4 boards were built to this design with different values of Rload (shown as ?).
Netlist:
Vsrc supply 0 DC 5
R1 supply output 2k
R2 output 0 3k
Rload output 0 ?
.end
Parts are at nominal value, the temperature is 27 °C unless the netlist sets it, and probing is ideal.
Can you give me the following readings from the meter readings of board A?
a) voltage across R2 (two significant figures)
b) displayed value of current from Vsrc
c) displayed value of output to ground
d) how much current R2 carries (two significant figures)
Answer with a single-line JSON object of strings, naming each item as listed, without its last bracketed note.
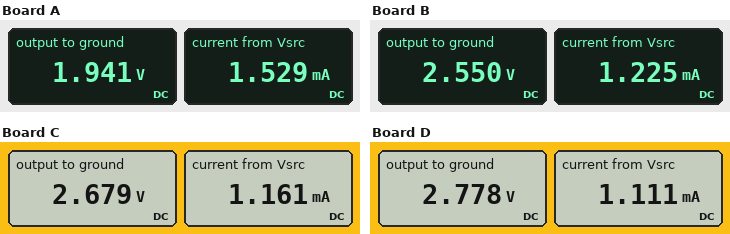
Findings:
{"voltage across R2": "1.9 V", "displayed value of current from Vsrc": "1.529 mA", "displayed value of output to ground": "1.941 V", "how much current R2 carries": "650 µA"}
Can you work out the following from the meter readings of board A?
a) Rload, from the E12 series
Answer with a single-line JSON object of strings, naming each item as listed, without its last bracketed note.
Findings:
{"Rload, from the E12 series": "2.2 kΩ"}
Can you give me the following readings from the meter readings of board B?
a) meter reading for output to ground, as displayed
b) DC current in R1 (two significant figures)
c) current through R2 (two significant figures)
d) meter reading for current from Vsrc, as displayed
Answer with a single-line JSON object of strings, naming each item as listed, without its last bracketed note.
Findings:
{"meter reading for output to ground, as displayed": "2.550 V", "DC current in R1": "1.2 mA", "current through R2": "850 µA", "meter reading for current from Vsrc, as displayed": "1.225 mA"}
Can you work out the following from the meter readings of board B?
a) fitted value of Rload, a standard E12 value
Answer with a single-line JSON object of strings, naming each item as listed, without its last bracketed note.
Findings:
{"fitted value of Rload, a standard E12 value": "6.8 kΩ"}
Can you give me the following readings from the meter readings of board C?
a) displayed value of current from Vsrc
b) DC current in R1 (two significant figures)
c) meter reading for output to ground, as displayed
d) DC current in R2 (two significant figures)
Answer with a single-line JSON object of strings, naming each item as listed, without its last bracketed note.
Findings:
{"displayed value of current from Vsrc": "1.161 mA", "DC current in R1": "1.2 mA", "meter reading for output to ground, as displayed": "2.679 V", "DC current in R2": "890 µA"}
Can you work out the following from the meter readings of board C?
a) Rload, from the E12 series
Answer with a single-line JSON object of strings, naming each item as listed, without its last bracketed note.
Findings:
{"Rload, from the E12 series": "10 kΩ"}
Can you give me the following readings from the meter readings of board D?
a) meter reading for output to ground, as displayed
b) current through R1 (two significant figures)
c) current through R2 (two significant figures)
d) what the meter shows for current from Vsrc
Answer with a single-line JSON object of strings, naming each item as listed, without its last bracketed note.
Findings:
{"meter reading for output to ground, as displayed": "2.778 V", "current through R1": "1.1 mA", "current through R2": "930 µA", "what the meter shows for current from Vsrc": "1.111 mA"}
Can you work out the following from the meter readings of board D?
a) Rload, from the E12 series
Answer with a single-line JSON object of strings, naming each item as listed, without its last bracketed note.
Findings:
{"Rload, from the E12 series": "15 kΩ"}
